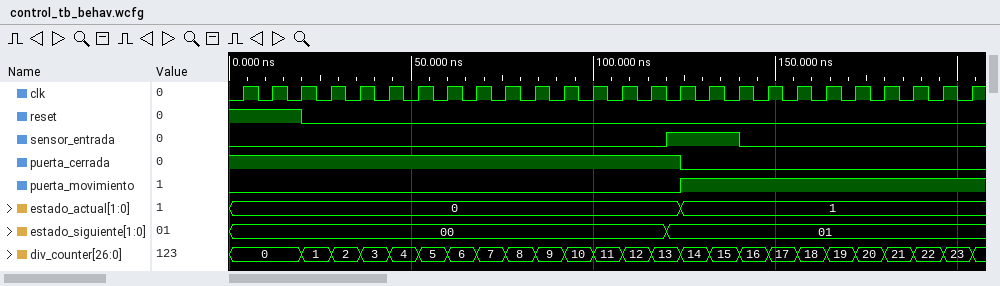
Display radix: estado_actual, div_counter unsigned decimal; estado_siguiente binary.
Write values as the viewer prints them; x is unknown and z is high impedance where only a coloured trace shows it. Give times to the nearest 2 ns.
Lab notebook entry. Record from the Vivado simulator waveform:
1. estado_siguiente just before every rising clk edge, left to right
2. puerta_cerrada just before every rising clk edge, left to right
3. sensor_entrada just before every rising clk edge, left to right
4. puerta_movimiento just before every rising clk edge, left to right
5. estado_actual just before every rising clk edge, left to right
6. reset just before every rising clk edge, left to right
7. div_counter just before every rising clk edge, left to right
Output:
00, 00, 00, 00, 00, 00, 00, 00, 00, 00, 00, 00, 00, 00, 00, 01, 01, 01, 01, 01, 01, 01, 01, 01, 01, 01
1 1 1 1 1 1 1 1 1 1 1 1 1 1 1 1 0 0 0 0 0 0 0 0 0 0
0 0 0 0 0 0 0 0 0 0 0 0 0 0 0 1 1 1 0 0 0 0 0 0 0 0
0 0 0 0 0 0 0 0 0 0 0 0 0 0 0 0 1 1 1 1 1 1 1 1 1 1
0, 0, 0, 0, 0, 0, 0, 0, 0, 0, 0, 0, 0, 0, 0, 0, 1, 1, 1, 1, 1, 1, 1, 1, 1, 1
1 1 1 0 0 0 0 0 0 0 0 0 0 0 0 0 0 0 0 0 0 0 0 0 0 0
0, 0, 0, 1, 2, 3, 4, 5, 6, 7, 8, 9, 10, 11, 12, 13, 14, 15, 16, 17, 18, 19, 20, 21, 22, 23
